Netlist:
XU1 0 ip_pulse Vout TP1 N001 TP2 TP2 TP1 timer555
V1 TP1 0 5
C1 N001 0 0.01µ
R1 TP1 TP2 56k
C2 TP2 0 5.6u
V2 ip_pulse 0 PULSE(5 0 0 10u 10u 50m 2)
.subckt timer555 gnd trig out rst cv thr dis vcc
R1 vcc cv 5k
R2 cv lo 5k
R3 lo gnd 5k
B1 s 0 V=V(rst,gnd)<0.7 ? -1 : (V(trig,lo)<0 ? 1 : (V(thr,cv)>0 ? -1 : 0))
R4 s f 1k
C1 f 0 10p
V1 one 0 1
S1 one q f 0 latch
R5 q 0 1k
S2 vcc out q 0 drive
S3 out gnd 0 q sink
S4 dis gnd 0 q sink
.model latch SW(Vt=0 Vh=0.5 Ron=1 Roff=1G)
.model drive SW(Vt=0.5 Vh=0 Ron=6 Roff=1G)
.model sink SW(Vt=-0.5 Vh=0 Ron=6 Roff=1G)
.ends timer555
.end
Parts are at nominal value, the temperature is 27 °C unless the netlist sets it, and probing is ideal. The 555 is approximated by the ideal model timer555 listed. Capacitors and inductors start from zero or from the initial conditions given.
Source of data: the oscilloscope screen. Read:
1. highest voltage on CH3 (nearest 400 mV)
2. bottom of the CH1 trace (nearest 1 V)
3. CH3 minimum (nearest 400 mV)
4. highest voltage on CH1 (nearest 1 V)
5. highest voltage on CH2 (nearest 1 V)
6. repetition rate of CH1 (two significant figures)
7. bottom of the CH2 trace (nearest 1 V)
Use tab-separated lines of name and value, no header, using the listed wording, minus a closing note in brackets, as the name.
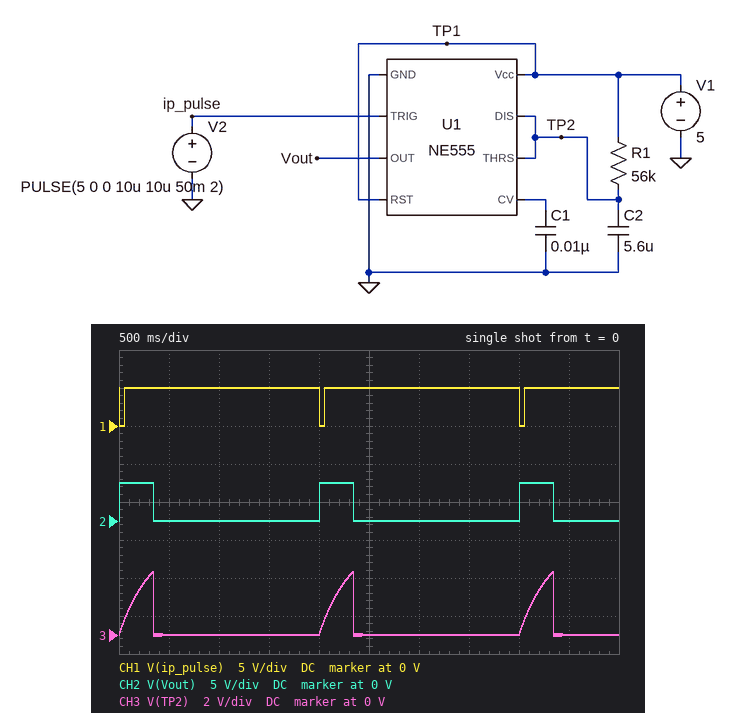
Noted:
highest voltage on CH3	3.2 V
bottom of the CH1 trace	0 V
CH3 minimum	0 V
highest voltage on CH1	5 V
highest voltage on CH2	5 V
repetition rate of CH1	500 mHz
bottom of the CH2 trace	0 V
